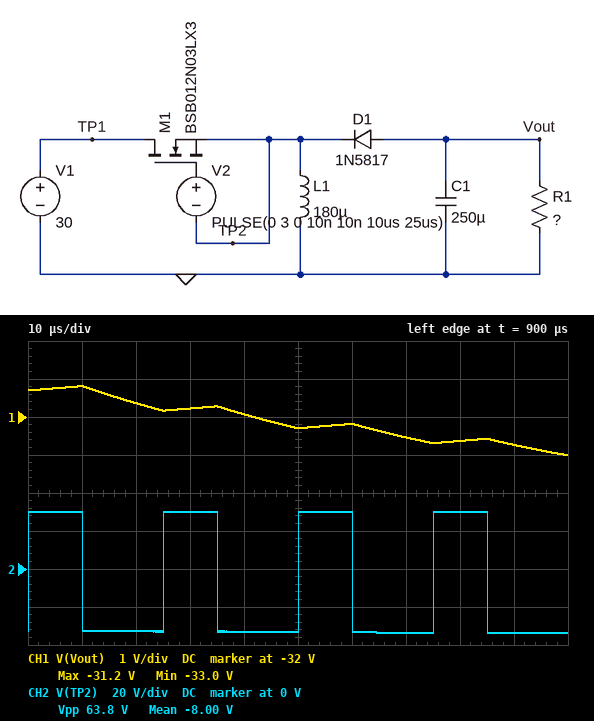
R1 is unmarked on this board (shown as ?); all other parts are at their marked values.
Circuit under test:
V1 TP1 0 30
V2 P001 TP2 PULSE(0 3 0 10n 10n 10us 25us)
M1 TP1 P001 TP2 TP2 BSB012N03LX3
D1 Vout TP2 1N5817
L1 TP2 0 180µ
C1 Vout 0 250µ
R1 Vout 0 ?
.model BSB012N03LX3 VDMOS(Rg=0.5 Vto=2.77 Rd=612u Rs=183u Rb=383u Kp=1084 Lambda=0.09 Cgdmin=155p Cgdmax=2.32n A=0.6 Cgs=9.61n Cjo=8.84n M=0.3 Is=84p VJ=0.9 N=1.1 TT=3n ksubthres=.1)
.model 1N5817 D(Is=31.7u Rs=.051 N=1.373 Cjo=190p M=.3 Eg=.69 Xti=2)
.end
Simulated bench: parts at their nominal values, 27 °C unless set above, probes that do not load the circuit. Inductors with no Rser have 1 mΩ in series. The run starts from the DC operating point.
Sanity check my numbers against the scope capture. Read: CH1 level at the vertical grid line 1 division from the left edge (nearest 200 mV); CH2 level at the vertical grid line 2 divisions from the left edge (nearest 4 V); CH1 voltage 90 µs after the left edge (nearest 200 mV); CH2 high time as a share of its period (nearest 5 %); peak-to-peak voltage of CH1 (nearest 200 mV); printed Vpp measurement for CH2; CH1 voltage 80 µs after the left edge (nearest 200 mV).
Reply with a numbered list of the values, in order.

1. -31.2 V
2. -32 V
3. -32.8 V
4. 40 %
5. 1.8 V
6. 63.8 V
7. -32.6 V
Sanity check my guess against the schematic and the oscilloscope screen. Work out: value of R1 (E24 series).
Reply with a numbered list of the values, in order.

1. 11 Ω
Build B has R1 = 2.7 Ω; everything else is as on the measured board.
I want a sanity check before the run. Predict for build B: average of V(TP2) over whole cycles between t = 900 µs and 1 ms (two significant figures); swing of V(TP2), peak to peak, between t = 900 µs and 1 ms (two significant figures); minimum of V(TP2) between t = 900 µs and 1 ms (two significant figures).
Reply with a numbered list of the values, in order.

1. -4.0 V
2. 57 V
3. -27 V
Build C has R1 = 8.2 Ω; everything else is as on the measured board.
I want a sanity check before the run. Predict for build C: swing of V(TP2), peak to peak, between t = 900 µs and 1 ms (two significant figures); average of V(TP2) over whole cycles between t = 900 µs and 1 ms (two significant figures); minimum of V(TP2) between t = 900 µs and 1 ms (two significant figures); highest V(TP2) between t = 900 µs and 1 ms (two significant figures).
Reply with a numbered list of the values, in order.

1. 63 V
2. -7.5 V
3. -33 V
4. 30 V
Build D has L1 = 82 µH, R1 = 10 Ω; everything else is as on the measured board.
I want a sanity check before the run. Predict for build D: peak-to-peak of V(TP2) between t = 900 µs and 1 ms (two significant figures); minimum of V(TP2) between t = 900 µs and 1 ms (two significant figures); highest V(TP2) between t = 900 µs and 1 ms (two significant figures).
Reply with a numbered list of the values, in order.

1. 62 V
2. -32 V
3. 30 V
